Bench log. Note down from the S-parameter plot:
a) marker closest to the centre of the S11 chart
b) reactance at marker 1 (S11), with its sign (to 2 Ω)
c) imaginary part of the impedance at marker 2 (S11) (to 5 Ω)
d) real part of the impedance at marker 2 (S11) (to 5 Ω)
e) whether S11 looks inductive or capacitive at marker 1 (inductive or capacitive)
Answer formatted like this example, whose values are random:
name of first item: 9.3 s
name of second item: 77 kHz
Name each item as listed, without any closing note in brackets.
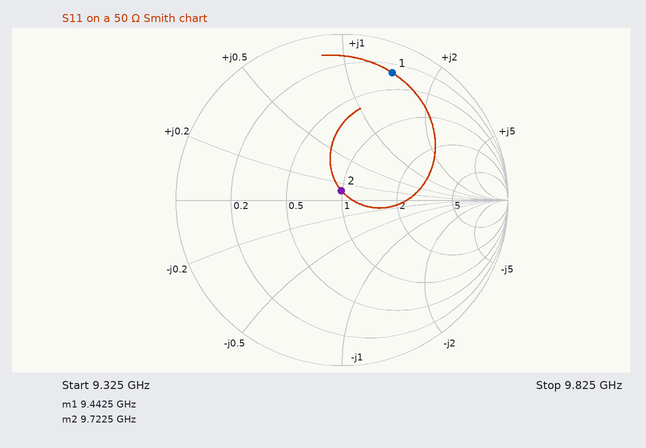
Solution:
marker closest to the centre of the S11 chart: marker 2
reactance at marker 1 (S11), with its sign: +72 Ω
imaginary part of the impedance at marker 2 (S11): +5 Ω
real part of the impedance at marker 2 (S11): 50 Ω
whether S11 looks inductive or capacitive at marker 1: inductive
